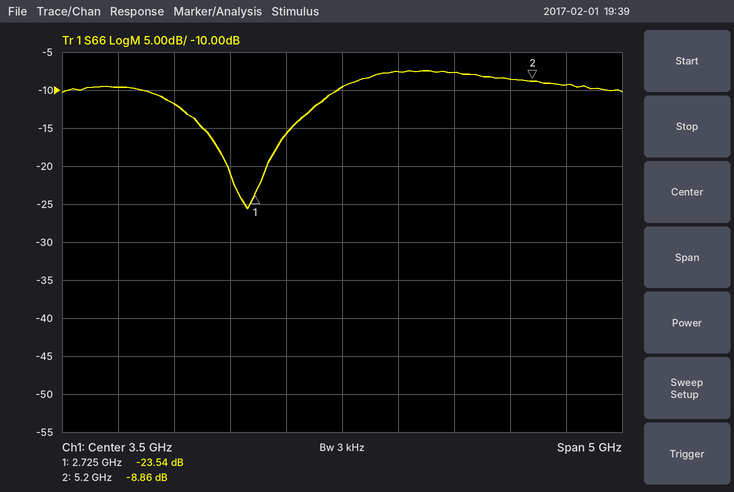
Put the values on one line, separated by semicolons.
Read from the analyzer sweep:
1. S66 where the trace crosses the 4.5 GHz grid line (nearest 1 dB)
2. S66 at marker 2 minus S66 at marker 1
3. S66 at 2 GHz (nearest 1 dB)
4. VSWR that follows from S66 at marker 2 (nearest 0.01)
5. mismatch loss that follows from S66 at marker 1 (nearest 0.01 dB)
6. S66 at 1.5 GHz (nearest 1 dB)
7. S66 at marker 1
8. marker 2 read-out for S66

-8 dB; 14.68 dB; -12 dB; 2.13; 0.02 dB; -10 dB; -23.54 dB; -8.86 dB
